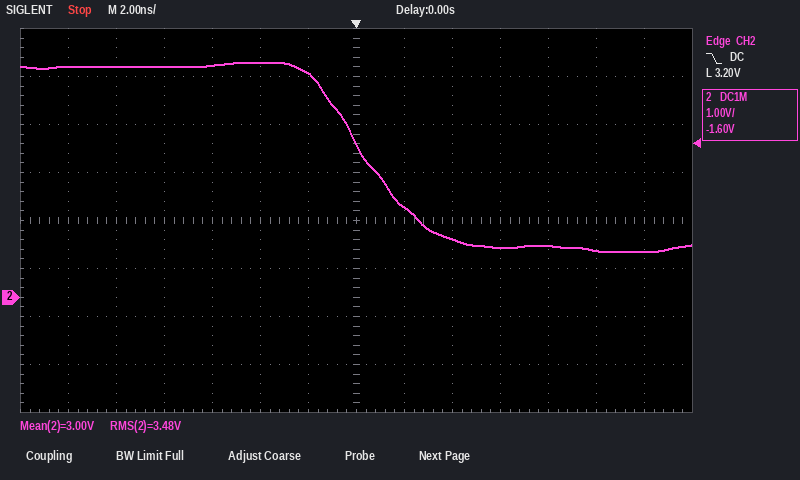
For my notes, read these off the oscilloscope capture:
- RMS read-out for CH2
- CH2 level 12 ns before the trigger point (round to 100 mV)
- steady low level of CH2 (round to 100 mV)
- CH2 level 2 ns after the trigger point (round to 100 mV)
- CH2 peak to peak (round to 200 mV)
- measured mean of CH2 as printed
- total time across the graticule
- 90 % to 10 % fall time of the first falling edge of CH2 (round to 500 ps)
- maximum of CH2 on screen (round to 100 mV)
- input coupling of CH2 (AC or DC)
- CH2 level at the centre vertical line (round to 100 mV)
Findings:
3.48 V
4.8 V
1.0 V
1.9 V
4.0 V
3.00 V
28 ns
4.5 ns
4.9 V
DC
3.2 V
